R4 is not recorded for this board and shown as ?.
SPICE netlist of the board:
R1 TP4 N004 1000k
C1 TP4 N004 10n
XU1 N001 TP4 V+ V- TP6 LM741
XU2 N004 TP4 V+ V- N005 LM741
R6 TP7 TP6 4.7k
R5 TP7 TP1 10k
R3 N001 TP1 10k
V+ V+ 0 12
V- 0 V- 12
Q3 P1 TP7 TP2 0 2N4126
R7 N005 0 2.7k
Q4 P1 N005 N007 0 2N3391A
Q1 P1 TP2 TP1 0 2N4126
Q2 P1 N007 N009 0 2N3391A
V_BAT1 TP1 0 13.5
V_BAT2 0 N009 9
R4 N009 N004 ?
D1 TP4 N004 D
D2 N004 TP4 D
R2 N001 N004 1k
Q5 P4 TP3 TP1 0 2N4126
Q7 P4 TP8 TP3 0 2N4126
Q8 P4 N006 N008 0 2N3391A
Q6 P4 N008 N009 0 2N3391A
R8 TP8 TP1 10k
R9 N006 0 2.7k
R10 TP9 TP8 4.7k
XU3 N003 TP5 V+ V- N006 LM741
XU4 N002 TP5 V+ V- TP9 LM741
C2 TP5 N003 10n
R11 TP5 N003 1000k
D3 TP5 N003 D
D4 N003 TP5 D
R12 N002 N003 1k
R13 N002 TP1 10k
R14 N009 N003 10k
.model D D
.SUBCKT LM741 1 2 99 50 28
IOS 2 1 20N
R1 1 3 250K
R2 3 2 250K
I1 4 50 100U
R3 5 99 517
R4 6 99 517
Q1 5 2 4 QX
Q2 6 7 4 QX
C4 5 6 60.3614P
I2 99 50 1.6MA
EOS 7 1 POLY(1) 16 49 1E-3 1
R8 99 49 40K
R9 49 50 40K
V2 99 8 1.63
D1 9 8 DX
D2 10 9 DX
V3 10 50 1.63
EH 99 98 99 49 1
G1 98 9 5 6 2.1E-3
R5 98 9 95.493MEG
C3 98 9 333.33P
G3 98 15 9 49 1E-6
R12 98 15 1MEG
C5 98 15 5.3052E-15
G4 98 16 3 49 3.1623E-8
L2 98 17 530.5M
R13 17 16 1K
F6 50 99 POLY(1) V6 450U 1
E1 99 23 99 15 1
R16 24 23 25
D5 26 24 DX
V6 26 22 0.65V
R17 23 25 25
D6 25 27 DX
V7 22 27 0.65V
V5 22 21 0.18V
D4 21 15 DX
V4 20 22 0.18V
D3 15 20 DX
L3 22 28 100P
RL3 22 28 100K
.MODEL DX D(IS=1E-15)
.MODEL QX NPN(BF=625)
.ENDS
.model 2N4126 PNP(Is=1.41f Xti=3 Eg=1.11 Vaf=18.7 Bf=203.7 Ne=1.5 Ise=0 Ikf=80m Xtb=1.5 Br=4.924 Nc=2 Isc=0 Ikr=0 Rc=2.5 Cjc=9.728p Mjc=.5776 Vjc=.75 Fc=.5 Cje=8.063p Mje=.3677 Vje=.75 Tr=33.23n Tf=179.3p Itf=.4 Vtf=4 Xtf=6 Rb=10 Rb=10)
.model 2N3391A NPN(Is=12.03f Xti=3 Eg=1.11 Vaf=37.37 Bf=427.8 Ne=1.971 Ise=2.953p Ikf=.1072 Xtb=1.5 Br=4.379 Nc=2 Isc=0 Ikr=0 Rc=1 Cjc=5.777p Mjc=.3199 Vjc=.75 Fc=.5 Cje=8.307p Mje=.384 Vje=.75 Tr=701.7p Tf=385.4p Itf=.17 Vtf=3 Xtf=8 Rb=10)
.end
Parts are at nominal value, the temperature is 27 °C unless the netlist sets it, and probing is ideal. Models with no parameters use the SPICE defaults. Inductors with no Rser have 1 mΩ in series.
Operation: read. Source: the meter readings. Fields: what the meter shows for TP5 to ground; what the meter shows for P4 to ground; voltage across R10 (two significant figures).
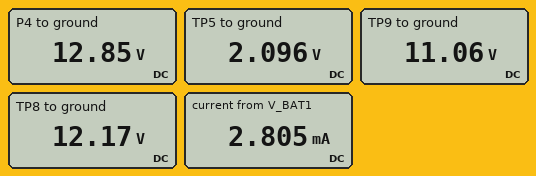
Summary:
2.096 V
12.85 V
1.1 V
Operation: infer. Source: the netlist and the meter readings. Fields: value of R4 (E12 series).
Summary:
6.8 kΩ
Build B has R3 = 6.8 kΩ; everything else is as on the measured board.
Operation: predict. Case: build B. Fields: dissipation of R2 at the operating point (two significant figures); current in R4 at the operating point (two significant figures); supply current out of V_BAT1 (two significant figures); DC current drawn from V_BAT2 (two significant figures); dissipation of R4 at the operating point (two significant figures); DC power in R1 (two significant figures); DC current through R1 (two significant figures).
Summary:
2.4 mW
1.5 mA
3.1 mA
2.6 mA
16 mW
210 nW
460 nA
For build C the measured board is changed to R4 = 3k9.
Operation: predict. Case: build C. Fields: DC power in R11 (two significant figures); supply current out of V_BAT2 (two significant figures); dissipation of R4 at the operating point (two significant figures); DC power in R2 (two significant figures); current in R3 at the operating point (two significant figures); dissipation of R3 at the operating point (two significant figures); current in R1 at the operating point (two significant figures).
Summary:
150 nW
2.6 mA
8.9 mW
2.3 mW
1.5 mA
23 mW
460 nA
